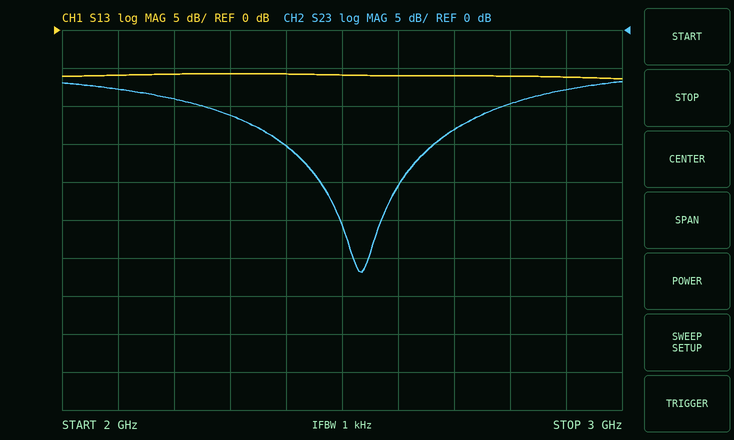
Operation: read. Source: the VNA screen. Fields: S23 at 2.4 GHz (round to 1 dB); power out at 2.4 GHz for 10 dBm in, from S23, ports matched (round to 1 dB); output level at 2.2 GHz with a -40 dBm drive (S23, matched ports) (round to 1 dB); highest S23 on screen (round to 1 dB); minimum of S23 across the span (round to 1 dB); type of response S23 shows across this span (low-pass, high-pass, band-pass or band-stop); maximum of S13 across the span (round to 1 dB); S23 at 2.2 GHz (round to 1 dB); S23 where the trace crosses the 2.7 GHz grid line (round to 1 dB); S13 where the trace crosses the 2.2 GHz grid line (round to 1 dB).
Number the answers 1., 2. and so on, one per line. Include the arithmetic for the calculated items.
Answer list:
1. -15 dB
2. 10 dBm + (-15 dB) = -5 dBm
3. -40 dBm + (-9 dB) = -49 dBm
4. -7 dB
5. -32 dB
6. band-stop
7. -6 dB
8. -9 dB
9. -13 dB
10. -6 dB
